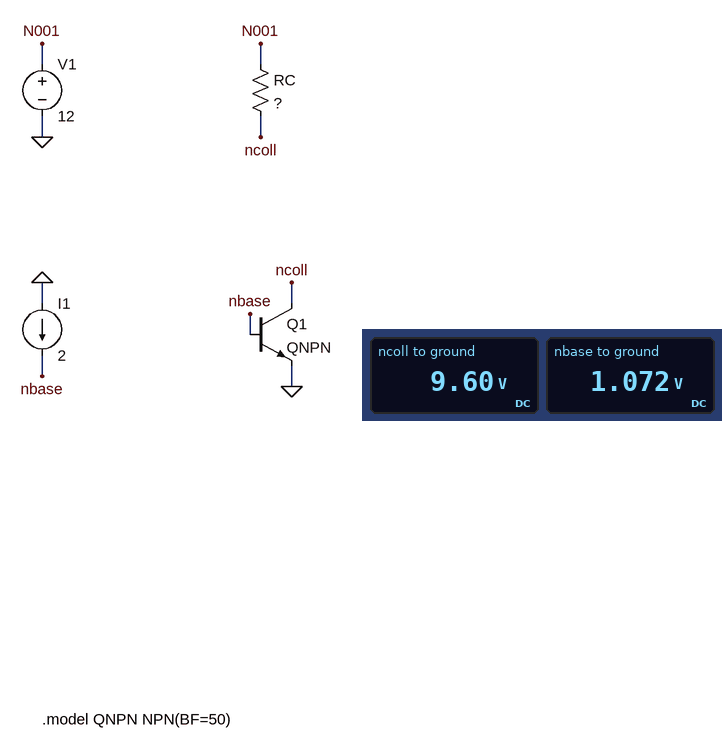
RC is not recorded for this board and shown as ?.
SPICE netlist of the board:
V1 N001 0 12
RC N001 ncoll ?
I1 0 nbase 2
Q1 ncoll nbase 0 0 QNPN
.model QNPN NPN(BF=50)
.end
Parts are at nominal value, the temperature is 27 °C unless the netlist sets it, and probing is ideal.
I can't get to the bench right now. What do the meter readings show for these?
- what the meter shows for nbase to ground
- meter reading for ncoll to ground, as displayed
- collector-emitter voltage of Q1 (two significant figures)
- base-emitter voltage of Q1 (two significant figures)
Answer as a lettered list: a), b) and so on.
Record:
a) 1.072 V
b) 9.60 V
c) 9.6 V
d) 1.1 V
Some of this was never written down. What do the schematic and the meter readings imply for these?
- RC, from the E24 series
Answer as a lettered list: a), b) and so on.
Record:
a) 0.024 Ω
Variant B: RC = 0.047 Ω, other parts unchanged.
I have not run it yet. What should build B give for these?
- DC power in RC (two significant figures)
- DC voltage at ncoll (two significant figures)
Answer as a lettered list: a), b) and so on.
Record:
a) 470 W
b) 7.3 V
